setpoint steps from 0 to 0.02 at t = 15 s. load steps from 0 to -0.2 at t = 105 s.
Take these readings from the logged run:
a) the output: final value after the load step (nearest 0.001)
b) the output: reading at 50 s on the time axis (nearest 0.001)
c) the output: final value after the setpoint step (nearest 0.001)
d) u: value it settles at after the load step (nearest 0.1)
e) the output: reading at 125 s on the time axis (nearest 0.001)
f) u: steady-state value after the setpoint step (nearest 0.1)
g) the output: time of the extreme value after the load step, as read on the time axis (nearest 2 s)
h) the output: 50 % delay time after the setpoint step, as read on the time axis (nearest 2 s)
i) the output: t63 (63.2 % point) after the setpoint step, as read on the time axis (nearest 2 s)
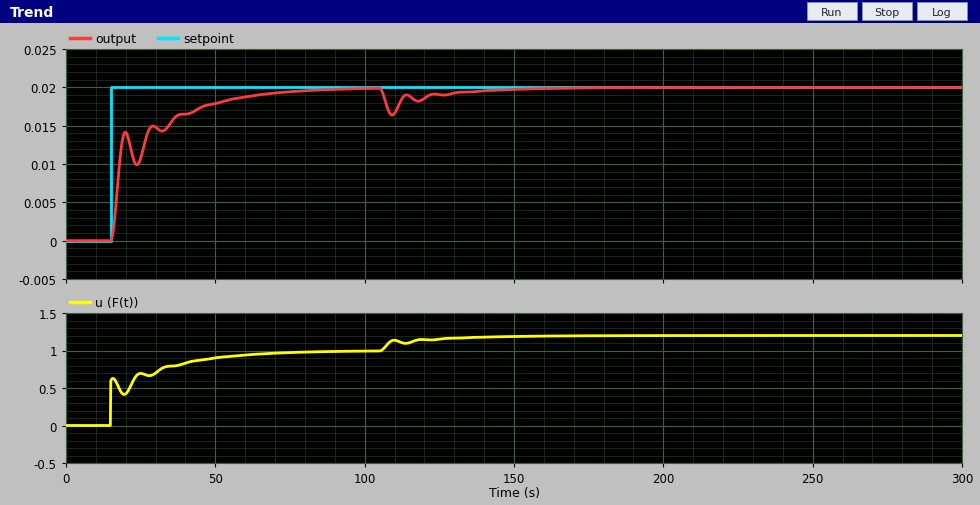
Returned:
0.020
0.018
0.020
1.2
0.019
1.0
110 s
18 s
18 s
